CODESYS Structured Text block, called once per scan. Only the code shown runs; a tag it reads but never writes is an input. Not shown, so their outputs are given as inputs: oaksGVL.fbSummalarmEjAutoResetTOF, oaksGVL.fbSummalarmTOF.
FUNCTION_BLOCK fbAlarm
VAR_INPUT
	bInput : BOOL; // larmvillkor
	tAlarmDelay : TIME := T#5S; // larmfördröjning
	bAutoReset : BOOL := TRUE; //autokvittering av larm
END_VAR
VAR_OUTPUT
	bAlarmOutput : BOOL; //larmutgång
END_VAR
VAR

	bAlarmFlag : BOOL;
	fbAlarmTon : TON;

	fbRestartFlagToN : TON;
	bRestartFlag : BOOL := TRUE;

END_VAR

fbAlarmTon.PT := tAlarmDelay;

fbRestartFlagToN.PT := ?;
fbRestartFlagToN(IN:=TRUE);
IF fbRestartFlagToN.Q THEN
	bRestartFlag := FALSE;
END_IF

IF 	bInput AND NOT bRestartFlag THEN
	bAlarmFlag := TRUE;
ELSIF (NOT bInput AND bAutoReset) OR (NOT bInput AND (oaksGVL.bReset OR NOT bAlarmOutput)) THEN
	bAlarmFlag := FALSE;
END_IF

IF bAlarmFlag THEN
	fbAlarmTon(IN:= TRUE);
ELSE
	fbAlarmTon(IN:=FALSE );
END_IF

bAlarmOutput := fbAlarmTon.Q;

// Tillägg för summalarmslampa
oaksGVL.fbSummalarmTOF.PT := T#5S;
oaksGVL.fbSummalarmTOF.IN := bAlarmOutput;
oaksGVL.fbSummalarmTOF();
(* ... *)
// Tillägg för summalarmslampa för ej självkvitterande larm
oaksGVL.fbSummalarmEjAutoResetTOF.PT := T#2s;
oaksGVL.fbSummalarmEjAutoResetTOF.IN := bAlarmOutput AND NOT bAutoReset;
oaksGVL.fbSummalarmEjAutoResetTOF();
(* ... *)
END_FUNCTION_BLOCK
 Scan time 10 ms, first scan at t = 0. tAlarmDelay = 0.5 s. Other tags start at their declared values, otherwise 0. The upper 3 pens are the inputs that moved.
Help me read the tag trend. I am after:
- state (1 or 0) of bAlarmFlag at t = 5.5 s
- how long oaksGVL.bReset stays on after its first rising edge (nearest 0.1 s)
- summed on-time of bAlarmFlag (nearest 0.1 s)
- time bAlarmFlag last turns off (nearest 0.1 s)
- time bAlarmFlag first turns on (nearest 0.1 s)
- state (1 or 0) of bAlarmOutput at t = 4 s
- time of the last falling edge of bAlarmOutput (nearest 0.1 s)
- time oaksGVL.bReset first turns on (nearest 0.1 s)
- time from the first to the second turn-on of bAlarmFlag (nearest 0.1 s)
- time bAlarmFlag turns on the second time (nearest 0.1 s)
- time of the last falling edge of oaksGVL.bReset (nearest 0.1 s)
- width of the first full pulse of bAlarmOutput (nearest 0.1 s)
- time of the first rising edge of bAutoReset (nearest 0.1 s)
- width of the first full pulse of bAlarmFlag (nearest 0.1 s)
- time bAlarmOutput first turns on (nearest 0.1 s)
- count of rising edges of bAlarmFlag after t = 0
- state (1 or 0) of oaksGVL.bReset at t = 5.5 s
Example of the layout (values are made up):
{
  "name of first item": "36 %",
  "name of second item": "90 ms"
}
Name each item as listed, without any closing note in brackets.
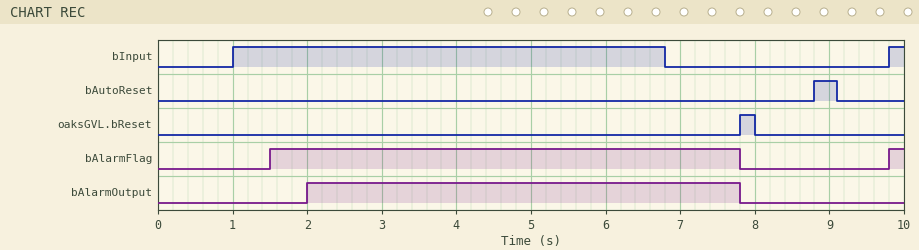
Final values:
{
  "state (1 or 0) of bAlarmFlag at t = 5.5 s": "1",
  "how long oaksGVL.bReset stays on after its first rising edge": "0.2 s",
  "summed on-time of bAlarmFlag": "6.5 s",
  "time bAlarmFlag last turns off": "7.8 s",
  "time bAlarmFlag first turns on": "1.5 s",
  "state (1 or 0) of bAlarmOutput at t = 4 s": "1",
  "time of the last falling edge of bAlarmOutput": "7.8 s",
  "time oaksGVL.bReset first turns on": "7.8 s",
  "time from the first to the second turn-on of bAlarmFlag": "8.3 s",
  "time bAlarmFlag turns on the second time": "9.8 s",
  "time of the last falling edge of oaksGVL.bReset": "8.0 s",
  "width of the first full pulse of bAlarmOutput": "5.8 s",
  "time of the first rising edge of bAutoReset": "8.8 s",
  "width of the first full pulse of bAlarmFlag": "6.3 s",
  "time bAlarmOutput first turns on": "2.0 s",
  "count of rising edges of bAlarmFlag after t = 0": "2",
  "state (1 or 0) of oaksGVL.bReset at t = 5.5 s": "0"
}
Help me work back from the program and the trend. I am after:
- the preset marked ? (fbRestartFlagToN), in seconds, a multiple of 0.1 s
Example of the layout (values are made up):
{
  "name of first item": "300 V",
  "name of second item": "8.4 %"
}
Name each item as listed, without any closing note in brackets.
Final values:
{
  "the preset marked ? (fbRestartFlagToN), in seconds, a multiple of 0.1 s": "1.5 s"
}
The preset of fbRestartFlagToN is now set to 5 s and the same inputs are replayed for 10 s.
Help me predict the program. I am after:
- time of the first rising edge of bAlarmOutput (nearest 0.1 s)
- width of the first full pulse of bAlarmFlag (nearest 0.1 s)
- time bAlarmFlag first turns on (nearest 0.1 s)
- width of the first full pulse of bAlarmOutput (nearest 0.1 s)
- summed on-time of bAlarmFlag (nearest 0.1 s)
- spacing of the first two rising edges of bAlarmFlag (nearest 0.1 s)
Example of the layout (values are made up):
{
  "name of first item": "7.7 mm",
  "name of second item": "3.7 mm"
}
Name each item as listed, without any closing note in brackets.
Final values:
{
  "time of the first rising edge of bAlarmOutput": "5.5 s",
  "width of the first full pulse of bAlarmFlag": "2.8 s",
  "time bAlarmFlag first turns on": "5.0 s",
  "width of the first full pulse of bAlarmOutput": "2.3 s",
  "summed on-time of bAlarmFlag": "3.0 s",
  "spacing of the first two rising edges of bAlarmFlag": "4.8 s"
}
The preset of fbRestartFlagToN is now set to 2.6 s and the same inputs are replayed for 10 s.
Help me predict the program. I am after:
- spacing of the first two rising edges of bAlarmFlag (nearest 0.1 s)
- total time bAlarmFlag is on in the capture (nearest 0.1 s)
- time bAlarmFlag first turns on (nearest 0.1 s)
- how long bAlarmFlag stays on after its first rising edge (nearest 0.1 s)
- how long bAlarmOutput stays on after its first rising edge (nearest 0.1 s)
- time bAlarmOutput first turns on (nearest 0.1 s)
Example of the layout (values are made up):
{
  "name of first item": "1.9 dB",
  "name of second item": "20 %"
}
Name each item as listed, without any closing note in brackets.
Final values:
{
  "spacing of the first two rising edges of bAlarmFlag": "7.2 s",
  "total time bAlarmFlag is on in the capture": "5.4 s",
  "time bAlarmFlag first turns on": "2.6 s",
  "how long bAlarmFlag stays on after its first rising edge": "5.2 s",
  "how long bAlarmOutput stays on after its first rising edge": "4.7 s",
  "time bAlarmOutput first turns on": "3.1 s"
}
